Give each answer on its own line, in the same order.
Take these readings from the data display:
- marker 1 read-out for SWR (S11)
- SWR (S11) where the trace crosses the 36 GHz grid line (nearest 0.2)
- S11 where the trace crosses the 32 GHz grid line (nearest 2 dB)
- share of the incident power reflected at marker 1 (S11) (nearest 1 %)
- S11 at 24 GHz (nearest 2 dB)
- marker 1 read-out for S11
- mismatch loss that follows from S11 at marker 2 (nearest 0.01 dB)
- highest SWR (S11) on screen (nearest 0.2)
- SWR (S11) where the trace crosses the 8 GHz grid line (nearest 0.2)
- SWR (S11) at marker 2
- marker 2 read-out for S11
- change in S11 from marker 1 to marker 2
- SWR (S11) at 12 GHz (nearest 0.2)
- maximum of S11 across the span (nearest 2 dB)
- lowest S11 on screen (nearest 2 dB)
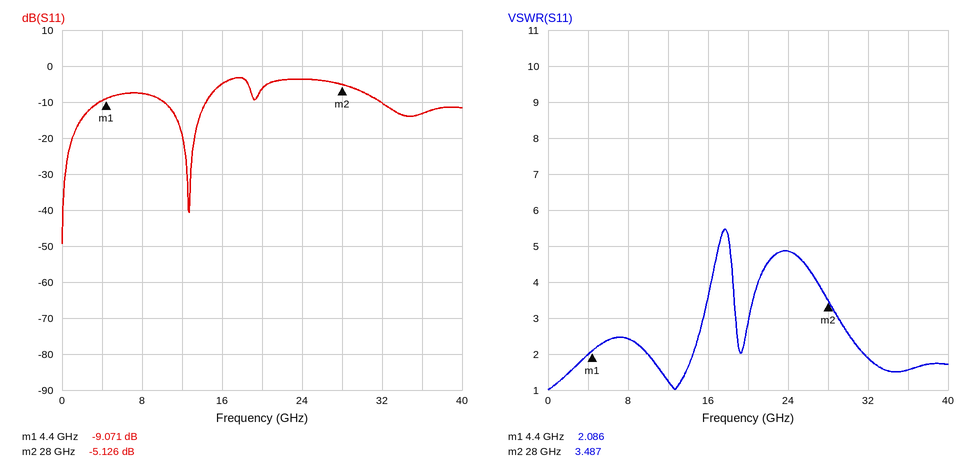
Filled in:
2.086
1.6
-10 dB
12 %
-4 dB
-9.071 dB
1.59 dB
5.4
2.4
3.487
-5.126 dB
3.945 dB
1.2
-4 dB
-50 dB
